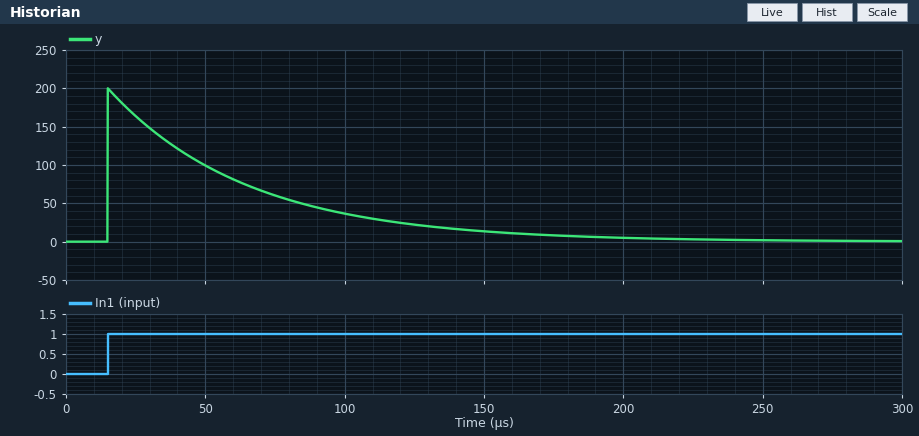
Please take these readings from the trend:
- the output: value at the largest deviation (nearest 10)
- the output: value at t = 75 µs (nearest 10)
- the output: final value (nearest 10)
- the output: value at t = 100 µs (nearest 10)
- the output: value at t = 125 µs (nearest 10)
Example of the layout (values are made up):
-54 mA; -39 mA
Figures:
200; 60; 0; 40; 20
